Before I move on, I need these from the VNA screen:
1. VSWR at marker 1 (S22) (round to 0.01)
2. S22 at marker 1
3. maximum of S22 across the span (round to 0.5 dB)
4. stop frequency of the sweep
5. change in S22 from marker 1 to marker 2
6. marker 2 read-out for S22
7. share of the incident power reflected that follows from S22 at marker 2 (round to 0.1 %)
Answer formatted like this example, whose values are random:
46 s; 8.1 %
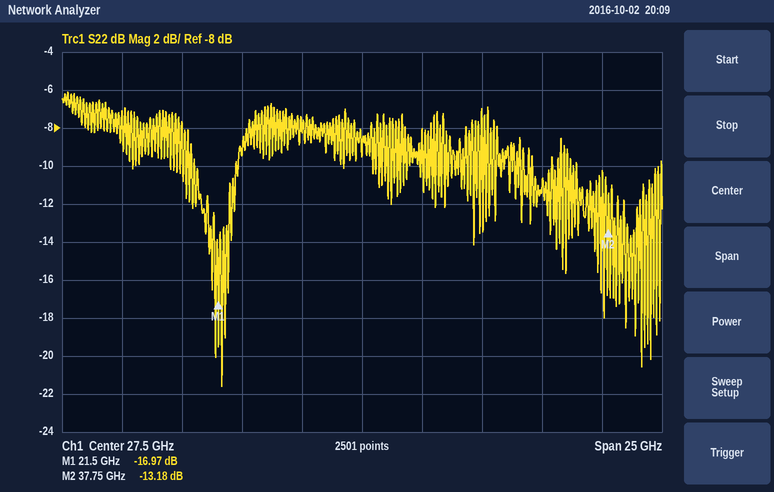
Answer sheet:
1.33; -16.97 dB; -6.0 dB; 40 GHz; 3.79 dB; -13.18 dB; 4.8 %
